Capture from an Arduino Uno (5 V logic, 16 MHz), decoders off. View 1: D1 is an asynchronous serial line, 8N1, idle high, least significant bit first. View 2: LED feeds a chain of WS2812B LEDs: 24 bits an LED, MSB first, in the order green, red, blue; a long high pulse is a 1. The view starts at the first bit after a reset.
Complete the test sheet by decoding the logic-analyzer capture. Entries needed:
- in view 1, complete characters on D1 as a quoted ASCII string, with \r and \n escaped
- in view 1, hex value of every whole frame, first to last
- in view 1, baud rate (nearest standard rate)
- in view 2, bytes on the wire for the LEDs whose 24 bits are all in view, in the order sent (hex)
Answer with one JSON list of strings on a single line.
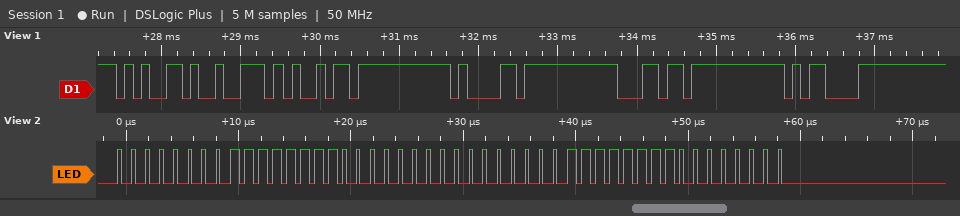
["\"erial\\r\"", "65 72 69 61 6C 0D", "9600 baud", "00 FF 00 00 FF 00"]
